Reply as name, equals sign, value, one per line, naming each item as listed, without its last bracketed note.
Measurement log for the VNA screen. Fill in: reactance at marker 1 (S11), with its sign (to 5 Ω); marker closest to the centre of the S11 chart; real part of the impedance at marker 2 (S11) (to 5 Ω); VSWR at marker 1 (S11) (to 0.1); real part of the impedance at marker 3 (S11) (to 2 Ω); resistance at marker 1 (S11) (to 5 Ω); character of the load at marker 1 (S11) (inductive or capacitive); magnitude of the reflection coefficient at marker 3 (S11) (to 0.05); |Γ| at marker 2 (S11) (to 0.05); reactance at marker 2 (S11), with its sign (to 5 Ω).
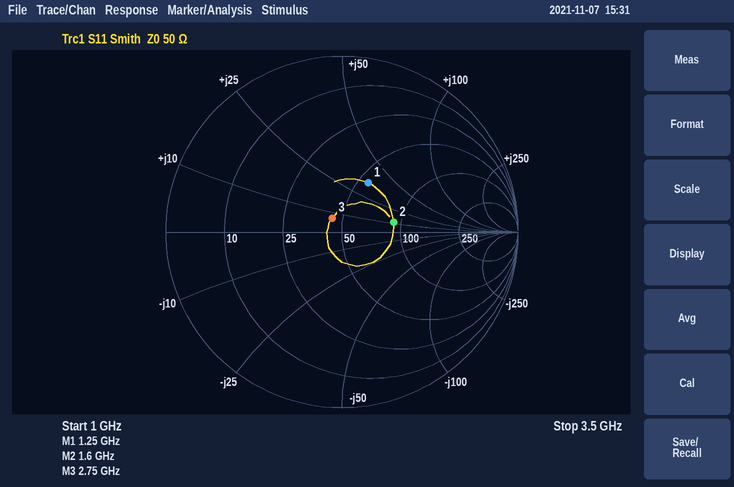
reactance at marker 1 (S11), with its sign = +35 Ω
marker closest to the centre of the S11 chart = marker 3
real part of the impedance at marker 2 (S11) = 90 Ω
VSWR at marker 1 (S11) = 1.9
real part of the impedance at marker 3 (S11) = 44 Ω
resistance at marker 1 (S11) = 55 Ω
character of the load at marker 1 (S11) = inductive
magnitude of the reflection coefficient at marker 3 (S11) = 0.10
|Γ| at marker 2 (S11) = 0.30
reactance at marker 2 (S11), with its sign = +10 Ω
